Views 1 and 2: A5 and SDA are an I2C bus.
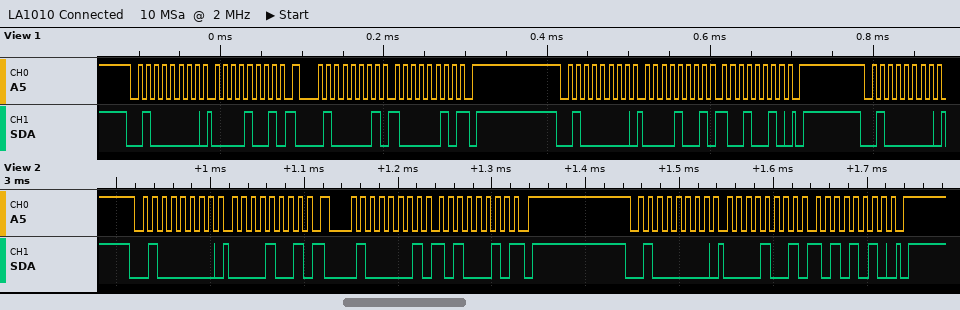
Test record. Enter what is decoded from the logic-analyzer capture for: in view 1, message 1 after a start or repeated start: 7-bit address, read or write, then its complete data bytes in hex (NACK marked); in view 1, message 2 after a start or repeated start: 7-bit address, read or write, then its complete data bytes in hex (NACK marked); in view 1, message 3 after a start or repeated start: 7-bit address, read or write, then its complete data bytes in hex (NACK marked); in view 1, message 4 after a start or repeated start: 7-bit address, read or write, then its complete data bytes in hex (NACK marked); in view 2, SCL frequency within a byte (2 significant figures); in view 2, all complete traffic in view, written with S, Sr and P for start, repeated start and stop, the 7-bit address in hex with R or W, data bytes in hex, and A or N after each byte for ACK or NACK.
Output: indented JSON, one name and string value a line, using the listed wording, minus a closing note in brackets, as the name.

{
  "in view 1, message 1 after a start or repeated start: 7-bit address, read or write, then its complete data bytes in hex": "0x20 write: 09",
  "in view 1, message 2 after a start or repeated start: 7-bit address, read or write, then its complete data bytes in hex": "0x20 read: 82 NACK",
  "in view 1, message 3 after a start or repeated start: 7-bit address, read or write, then its complete data bytes in hex": "0x20 write: 09 92",
  "in view 1, message 4 after a start or repeated start: 7-bit address, read or write, then its complete data bytes in hex": "0x20 write",
  "in view 2, SCL frequency within a byte": "100 kHz",
  "in view 2, all complete traffic in view, written with S, Sr and P for start, repeated start and stop, the 7-bit address in hex with R or W, data bytes in hex, and A or N after each byte for ACK or NACK": "S 20W A 09 A Sr 20R A A2 N P S 20W A 09 A AA A P"
}
